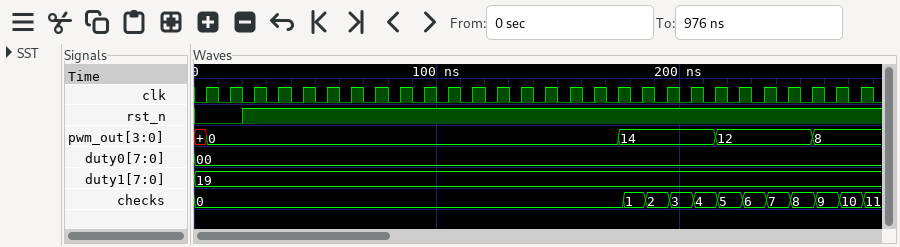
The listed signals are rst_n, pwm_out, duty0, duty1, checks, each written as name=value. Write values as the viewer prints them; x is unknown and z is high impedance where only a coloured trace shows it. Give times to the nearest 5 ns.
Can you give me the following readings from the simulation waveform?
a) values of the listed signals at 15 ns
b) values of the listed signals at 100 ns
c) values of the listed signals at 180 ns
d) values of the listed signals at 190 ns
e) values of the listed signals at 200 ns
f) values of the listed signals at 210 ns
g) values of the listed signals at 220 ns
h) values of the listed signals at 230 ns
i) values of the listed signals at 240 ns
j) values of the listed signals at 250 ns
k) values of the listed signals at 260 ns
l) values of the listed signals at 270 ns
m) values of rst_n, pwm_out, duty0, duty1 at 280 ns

rst_n=0, pwm_out=0, duty0=00, duty1=19, checks=0
rst_n=1, pwm_out=0, duty0=00, duty1=19, checks=0
rst_n=1, pwm_out=14, duty0=00, duty1=19, checks=1
rst_n=1, pwm_out=14, duty0=00, duty1=19, checks=2
rst_n=1, pwm_out=14, duty0=00, duty1=19, checks=3
rst_n=1, pwm_out=14, duty0=00, duty1=19, checks=4
rst_n=1, pwm_out=12, duty0=00, duty1=19, checks=5
rst_n=1, pwm_out=12, duty0=00, duty1=19, checks=6
rst_n=1, pwm_out=12, duty0=00, duty1=19, checks=7
rst_n=1, pwm_out=12, duty0=00, duty1=19, checks=8
rst_n=1, pwm_out=8, duty0=00, duty1=19, checks=9
rst_n=1, pwm_out=8, duty0=00, duty1=19, checks=10
rst_n=1, pwm_out=8, duty0=00, duty1=19
